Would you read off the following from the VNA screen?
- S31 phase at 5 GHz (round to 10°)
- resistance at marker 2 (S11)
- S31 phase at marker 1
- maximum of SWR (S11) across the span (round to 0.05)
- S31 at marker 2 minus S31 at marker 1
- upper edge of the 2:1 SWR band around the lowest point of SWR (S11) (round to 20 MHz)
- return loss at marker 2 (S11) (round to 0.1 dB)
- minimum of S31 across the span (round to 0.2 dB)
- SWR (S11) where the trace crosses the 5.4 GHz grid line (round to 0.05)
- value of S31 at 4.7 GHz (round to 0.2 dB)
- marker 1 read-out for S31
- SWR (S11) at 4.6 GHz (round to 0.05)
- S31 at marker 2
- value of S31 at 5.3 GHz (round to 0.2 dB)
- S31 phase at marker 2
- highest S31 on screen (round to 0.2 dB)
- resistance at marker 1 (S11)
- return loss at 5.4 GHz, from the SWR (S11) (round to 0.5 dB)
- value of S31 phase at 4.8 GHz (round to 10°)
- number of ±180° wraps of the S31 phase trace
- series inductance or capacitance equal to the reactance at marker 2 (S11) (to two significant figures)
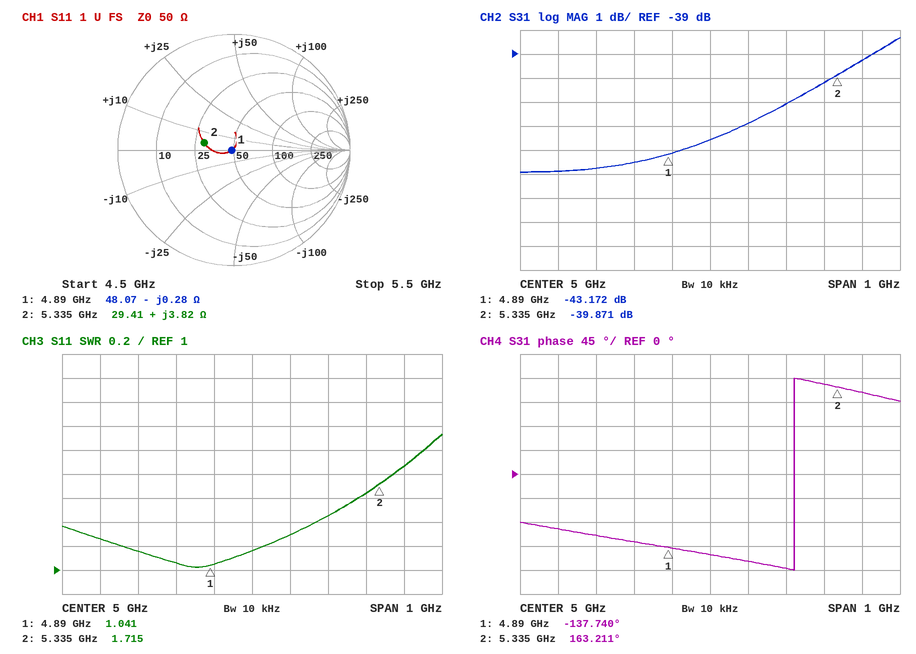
-150°
29.41 Ω
-137.740°
2.15
3.301 dB
5.46 GHz
11.6 dB
-44.0 dB
1.85
-43.8 dB
-43.172 dB
1.25
-39.871 dB
-40.2 dB
163.211°
-38.4 dB
48.07 Ω
10.5 dB
-130°
1
110 pH
